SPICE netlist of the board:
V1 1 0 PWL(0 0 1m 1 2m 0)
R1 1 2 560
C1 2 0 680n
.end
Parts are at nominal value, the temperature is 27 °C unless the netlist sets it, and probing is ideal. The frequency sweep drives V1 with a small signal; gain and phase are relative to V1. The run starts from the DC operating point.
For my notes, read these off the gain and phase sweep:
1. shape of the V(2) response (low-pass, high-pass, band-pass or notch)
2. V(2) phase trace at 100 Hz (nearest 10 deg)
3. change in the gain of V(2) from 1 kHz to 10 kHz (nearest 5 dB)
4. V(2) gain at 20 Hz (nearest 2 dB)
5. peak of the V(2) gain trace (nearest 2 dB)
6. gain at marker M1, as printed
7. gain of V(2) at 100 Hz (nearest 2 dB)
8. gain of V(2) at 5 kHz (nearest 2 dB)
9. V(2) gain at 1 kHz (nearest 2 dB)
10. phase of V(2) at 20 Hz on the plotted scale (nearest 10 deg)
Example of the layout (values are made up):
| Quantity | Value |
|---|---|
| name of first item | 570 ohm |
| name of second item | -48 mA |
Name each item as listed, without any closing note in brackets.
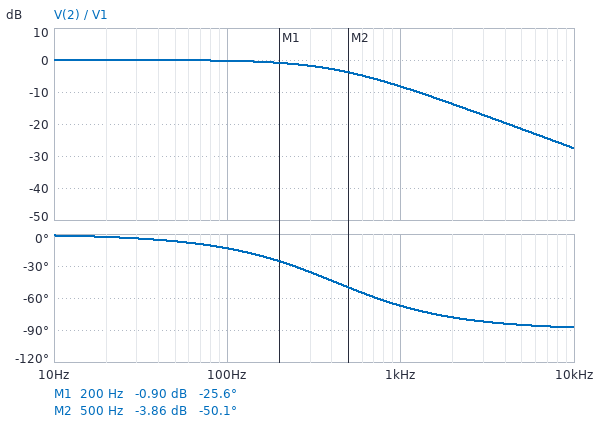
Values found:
| Quantity | Value |
|---|---|
| shape of the V(2) response | low-pass |
| V(2) phase trace at 100 Hz | -10 deg |
| change in the gain of V(2) from 1 kHz to 10 kHz | -20 dB |
| V(2) gain at 20 Hz | 0 dB |
| peak of the V(2) gain trace | 0 dB |
| gain at marker M1, as printed | -0.90 dB |
| gain of V(2) at 100 Hz | 0 dB |
| gain of V(2) at 5 kHz | -22 dB |
| V(2) gain at 1 kHz | -8 dB |
| phase of V(2) at 20 Hz on the plotted scale | 0 deg |
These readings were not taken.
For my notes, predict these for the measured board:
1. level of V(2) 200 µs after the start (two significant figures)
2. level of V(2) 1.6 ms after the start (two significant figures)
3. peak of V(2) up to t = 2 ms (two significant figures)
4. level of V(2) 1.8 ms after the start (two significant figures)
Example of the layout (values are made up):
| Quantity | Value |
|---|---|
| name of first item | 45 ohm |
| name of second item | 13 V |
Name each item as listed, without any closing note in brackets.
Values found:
| Quantity | Value |
|---|---|
| level of V(2) 200 µs after the start | 44 mV |
| level of V(2) 1.6 ms after the start | 630 mV |
| peak of V(2) up to t = 2 ms | 750 mV |
| level of V(2) 1.8 ms after the start | 490 mV |
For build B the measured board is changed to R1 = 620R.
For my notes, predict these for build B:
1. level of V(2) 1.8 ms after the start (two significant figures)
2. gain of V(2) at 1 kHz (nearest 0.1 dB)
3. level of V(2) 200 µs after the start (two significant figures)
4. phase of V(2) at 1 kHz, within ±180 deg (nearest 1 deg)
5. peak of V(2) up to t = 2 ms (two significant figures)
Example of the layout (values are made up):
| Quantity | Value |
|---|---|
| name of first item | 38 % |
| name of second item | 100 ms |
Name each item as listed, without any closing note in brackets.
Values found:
| Quantity | Value |
|---|---|
| level of V(2) 1.8 ms after the start | 500 mV |
| gain of V(2) at 1 kHz | -9.0 dB |
| level of V(2) 200 µs after the start | 41 mV |
| phase of V(2) at 1 kHz, within ±180 deg | -69 deg |
| peak of V(2) up to t = 2 ms | 730 mV |
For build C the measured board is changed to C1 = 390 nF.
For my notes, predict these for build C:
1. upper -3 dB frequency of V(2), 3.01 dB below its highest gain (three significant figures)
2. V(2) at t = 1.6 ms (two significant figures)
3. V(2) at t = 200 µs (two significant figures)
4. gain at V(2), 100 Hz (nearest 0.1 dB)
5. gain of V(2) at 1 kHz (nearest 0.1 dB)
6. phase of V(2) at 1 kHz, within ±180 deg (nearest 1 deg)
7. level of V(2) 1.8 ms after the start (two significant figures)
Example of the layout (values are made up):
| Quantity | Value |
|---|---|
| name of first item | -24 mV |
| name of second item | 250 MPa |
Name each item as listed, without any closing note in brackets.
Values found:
| Quantity | Value |
|---|---|
| upper -3 dB frequency of V(2), 3.01 dB below its highest gain | 729 Hz |
| V(2) at t = 1.6 ms | 590 mV |
| V(2) at t = 200 µs | 69 mV |
| gain at V(2), 100 Hz | -0.1 dB |
| gain of V(2) at 1 kHz | -4.6 dB |
| phase of V(2) at 1 kHz, within ±180 deg | -54 deg |
| level of V(2) 1.8 ms after the start | 410 mV |
